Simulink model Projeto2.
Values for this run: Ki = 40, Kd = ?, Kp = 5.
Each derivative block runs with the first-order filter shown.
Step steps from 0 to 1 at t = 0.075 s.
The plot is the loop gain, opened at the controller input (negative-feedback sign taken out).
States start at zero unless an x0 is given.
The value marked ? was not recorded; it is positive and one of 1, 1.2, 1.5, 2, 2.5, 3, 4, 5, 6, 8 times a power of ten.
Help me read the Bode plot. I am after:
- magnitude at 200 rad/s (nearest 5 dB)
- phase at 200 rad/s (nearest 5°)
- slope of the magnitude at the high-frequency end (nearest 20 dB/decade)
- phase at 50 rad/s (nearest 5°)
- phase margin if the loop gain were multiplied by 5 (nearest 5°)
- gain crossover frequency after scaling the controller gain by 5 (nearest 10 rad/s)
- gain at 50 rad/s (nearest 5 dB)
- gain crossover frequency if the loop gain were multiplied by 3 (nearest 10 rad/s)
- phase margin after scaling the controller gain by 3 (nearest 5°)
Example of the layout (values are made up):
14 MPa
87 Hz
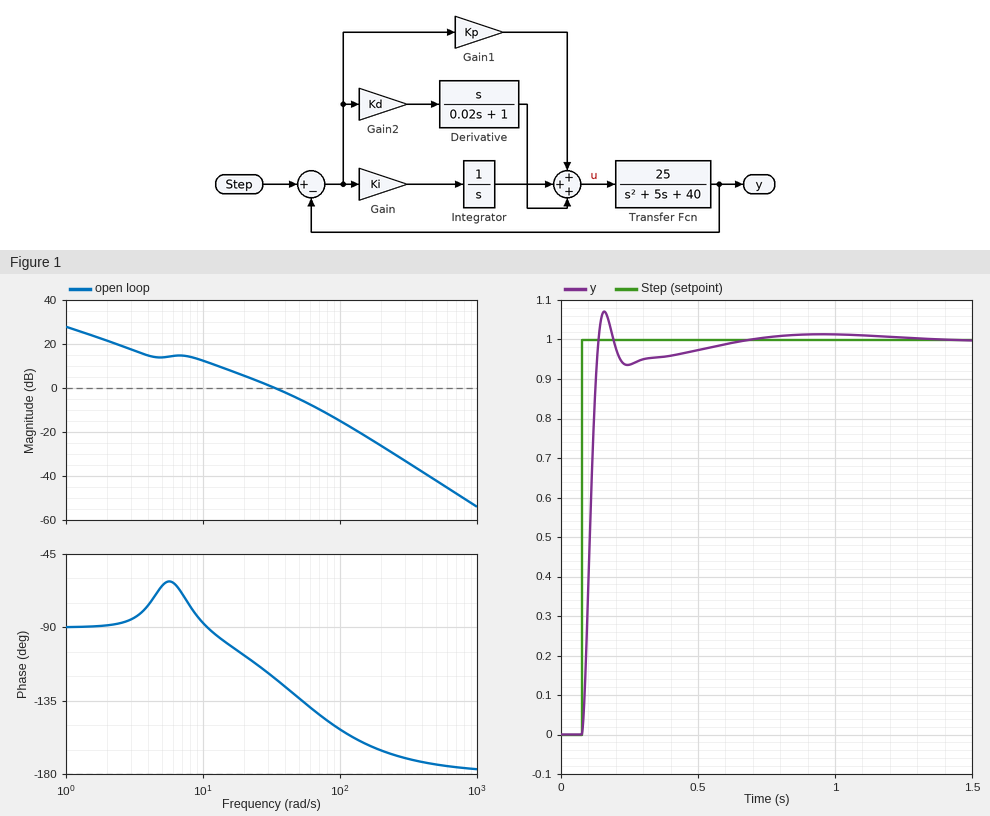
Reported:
-25 dB
-165°
-40 dB/decade
-135°
30°
90 rad/s
-5 dB
70 rad/s
35°
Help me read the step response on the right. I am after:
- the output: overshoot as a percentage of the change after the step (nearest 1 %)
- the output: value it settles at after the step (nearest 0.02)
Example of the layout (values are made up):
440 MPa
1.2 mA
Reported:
7 %
1.00
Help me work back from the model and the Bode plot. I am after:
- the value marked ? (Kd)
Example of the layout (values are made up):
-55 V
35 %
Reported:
1.5
